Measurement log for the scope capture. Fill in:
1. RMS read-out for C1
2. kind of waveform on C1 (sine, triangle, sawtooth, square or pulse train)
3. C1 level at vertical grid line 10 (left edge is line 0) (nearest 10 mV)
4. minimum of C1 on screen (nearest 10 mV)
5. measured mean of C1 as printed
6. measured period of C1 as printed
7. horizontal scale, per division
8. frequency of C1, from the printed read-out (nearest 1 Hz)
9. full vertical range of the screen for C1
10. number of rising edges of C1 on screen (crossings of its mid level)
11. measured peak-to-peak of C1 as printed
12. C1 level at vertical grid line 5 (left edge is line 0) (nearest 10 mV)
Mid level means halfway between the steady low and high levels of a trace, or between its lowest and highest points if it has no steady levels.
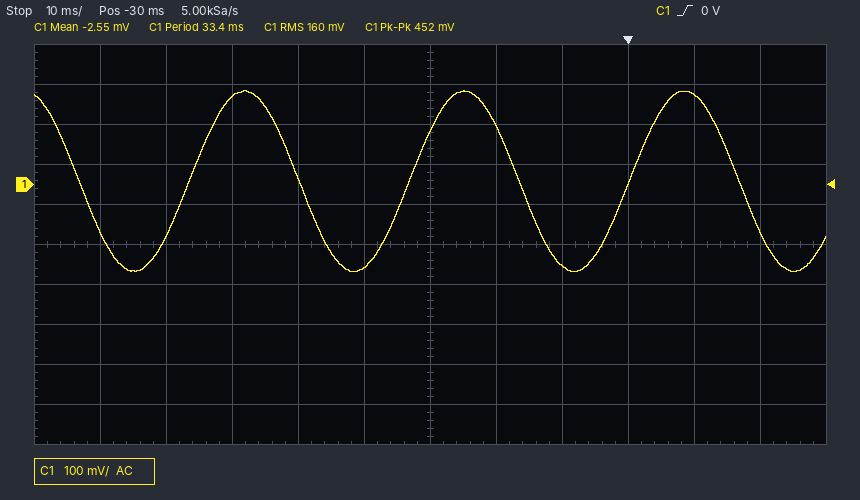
160 mV
sine
220 mV
-220 mV
-2.55 mV
33.4 ms
10 ms
30 Hz
1 V
3
452 mV
-210 mV
